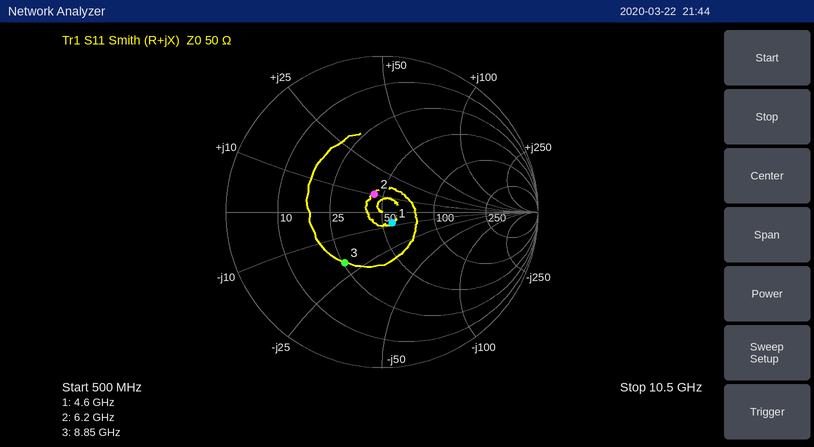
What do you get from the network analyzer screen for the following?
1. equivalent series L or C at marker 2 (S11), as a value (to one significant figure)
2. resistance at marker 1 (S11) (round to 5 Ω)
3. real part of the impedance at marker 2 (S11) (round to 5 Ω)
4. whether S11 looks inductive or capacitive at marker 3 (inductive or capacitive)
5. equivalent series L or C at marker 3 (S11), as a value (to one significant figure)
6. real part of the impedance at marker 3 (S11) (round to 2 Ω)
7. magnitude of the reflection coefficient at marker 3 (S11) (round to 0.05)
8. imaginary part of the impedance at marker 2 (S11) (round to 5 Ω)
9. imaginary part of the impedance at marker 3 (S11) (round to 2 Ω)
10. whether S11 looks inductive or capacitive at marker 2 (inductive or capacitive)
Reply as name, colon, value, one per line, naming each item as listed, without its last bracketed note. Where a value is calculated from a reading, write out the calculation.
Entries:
equivalent series L or C at marker 2 (S11), as a value: L = 10 Ω/(2π × 6.2 GHz) ≈ 257 pH, so 300 pH to one significant figure
resistance at marker 1 (S11): 55 Ω
real part of the impedance at marker 2 (S11): 45 Ω
whether S11 looks inductive or capacitive at marker 3: capacitive
equivalent series L or C at marker 3 (S11), as a value: C = 1/(2π × 8.85 GHz × 20 Ω) ≈ 899 fF, so 900 fF to one significant figure
real part of the impedance at marker 3 (S11): 26 Ω
magnitude of the reflection coefficient at marker 3 (S11): 0.40
imaginary part of the impedance at marker 2 (S11): +10 Ω
imaginary part of the impedance at marker 3 (S11): -20 Ω
whether S11 looks inductive or capacitive at marker 2: inductive
